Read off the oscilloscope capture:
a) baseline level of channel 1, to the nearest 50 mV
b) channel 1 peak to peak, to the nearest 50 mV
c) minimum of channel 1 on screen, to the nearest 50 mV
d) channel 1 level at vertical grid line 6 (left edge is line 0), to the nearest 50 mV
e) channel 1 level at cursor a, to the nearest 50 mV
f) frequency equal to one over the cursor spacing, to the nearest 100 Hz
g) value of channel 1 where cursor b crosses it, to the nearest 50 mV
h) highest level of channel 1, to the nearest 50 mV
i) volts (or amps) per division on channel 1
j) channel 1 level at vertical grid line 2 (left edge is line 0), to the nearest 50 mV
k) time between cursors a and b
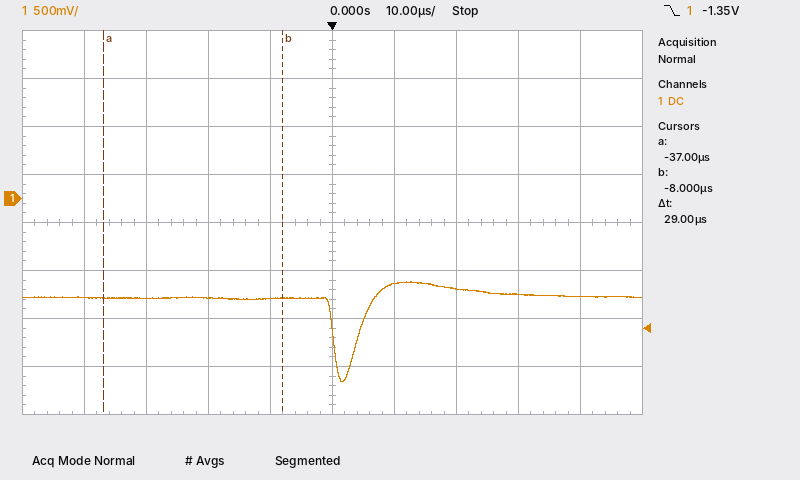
-1.05 V
1.05 V
-1.90 V
-900 mV
-1.05 V
34.5 kHz
-1.05 V
-850 mV
500 mV
-1.05 V
29 µs
